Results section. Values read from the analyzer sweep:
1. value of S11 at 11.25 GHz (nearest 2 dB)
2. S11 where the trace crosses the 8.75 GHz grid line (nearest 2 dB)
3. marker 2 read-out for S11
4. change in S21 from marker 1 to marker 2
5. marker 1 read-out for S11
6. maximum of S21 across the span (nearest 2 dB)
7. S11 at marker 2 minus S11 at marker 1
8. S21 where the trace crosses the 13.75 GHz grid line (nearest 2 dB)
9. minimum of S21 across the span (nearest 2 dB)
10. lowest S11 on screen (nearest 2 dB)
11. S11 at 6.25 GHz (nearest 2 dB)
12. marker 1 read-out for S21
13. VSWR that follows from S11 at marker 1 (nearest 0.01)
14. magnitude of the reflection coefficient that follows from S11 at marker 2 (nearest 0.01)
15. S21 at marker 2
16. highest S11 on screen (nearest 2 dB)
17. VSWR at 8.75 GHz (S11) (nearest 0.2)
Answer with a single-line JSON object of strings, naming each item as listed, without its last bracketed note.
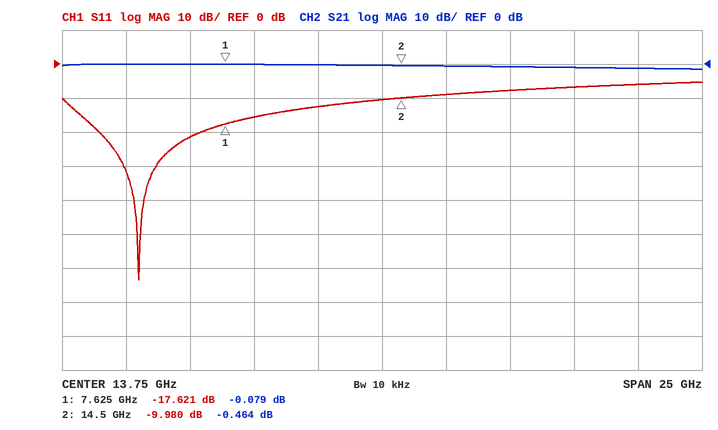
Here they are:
{"value of S11 at 11.25 GHz": "-12 dB", "S11 where the trace crosses the 8.75 GHz grid line": "-16 dB", "marker 2 read-out for S11": "-9.980 dB", "change in S21 from marker 1 to marker 2": "-0.385 dB", "marker 1 read-out for S11": "-17.621 dB", "maximum of S21 across the span": "0 dB", "S11 at marker 2 minus S11 at marker 1": "7.641 dB", "S21 where the trace crosses the 13.75 GHz grid line": "0 dB", "minimum of S21 across the span": "-2 dB", "lowest S11 on screen": "-64 dB", "S11 at 6.25 GHz": "-22 dB", "marker 1 read-out for S21": "-0.079 dB", "VSWR that follows from S11 at marker 1": "1.30", "magnitude of the reflection coefficient that follows from S11 at marker 2": "0.32", "S21 at marker 2": "-0.464 dB", "highest S11 on screen": "-6 dB", "VSWR at 8.75 GHz (S11)": "1.4"}
